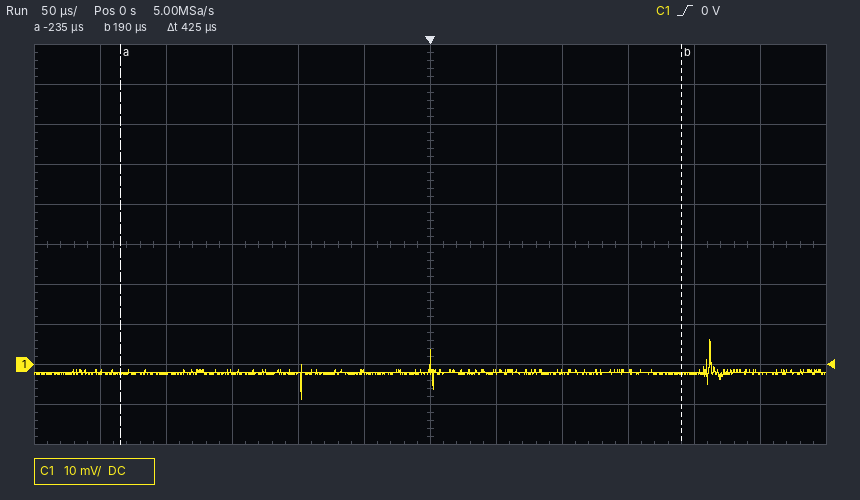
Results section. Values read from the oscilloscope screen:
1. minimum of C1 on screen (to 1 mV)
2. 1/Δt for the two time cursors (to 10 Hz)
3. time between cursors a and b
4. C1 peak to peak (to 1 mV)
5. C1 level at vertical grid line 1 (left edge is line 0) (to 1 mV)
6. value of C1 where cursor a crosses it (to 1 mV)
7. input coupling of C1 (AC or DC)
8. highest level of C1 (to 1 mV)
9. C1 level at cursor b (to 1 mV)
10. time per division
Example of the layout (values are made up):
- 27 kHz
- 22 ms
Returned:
- -9 mV
- 2.35 kHz
- 425 µs
- 15 mV
- -2 mV
- -2 mV
- DC
- 6 mV
- -2 mV
- 50 µs
